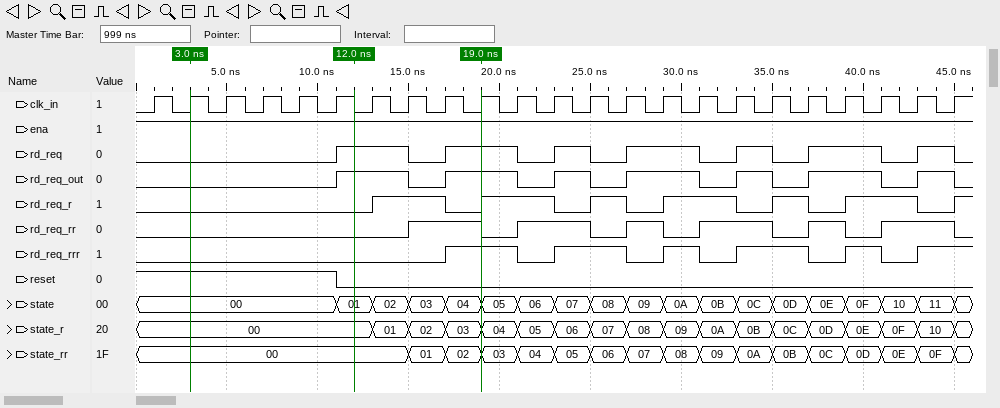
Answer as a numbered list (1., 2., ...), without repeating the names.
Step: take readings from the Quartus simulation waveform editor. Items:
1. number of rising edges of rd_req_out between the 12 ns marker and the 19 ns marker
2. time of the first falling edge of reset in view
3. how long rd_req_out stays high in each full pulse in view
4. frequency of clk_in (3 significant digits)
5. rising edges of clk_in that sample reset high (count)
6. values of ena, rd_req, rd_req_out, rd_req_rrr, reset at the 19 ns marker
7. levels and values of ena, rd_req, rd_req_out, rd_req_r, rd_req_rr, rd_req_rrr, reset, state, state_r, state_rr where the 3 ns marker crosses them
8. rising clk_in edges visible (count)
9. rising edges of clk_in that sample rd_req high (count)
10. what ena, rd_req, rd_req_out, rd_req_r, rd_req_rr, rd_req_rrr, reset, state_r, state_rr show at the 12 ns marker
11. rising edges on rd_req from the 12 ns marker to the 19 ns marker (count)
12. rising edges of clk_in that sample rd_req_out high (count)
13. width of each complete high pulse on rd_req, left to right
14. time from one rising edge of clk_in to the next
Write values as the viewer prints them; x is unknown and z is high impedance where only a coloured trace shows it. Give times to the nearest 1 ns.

1. 1
2. 11 ns
3. 4 ns, 4 ns, 2 ns, 4 ns, 2 ns, 4 ns, 2 ns
4. 500 MHz
5. 6
6. ena=1, rd_req=1, rd_req_out=1, rd_req_rrr=1, reset=0
7. ena=1, rd_req=0, rd_req_out=0, rd_req_r=0, rd_req_rr=0, rd_req_rrr=0, reset=1, state=00, state_r=00, state_rr=00
8. 23
9. 11
10. ena=1, rd_req=1, rd_req_out=1, rd_req_r=0, rd_req_rr=0, rd_req_rrr=0, reset=0, state_r=00, state_rr=00
11. 1
12. 11
13. 4 ns, 4 ns, 2 ns, 4 ns, 2 ns, 4 ns, 2 ns
14. 2 ns
